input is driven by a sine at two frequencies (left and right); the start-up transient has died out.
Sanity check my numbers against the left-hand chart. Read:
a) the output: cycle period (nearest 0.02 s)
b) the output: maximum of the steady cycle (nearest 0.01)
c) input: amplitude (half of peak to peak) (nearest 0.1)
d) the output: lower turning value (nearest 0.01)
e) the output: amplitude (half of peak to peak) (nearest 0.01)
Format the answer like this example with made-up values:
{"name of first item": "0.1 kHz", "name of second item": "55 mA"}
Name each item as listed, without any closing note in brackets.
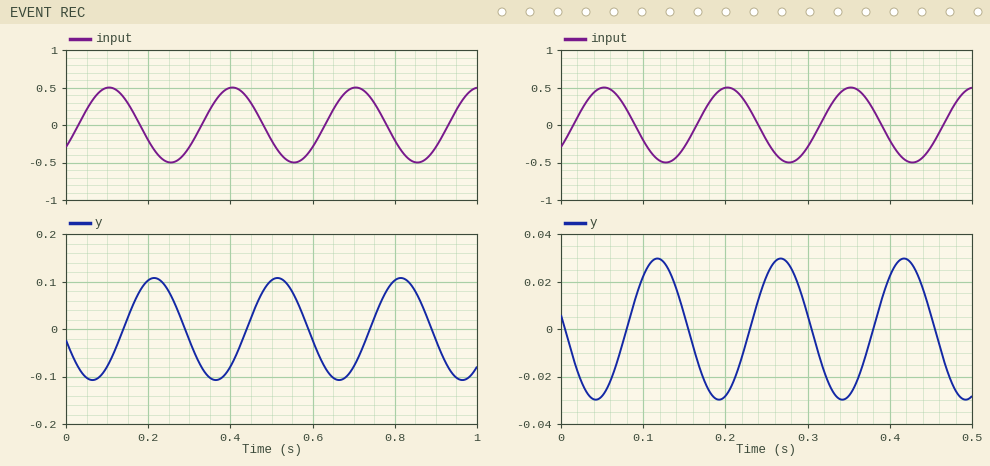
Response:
{"the output: cycle period": "0.30 s", "the output: maximum of the steady cycle": "0.11", "input: amplitude (half of peak to peak)": "0.5", "the output: lower turning value": "-0.11", "the output: amplitude (half of peak to peak)": "0.11"}
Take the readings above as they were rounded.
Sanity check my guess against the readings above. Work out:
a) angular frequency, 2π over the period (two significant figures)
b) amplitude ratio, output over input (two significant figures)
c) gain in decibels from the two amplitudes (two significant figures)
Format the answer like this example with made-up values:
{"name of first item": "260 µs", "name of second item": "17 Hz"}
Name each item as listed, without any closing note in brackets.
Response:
{"angular frequency, 2π over the period": "21 rad/s", "amplitude ratio, output over input": "0.22", "gain in decibels from the two amplitudes": "-13 dB"}
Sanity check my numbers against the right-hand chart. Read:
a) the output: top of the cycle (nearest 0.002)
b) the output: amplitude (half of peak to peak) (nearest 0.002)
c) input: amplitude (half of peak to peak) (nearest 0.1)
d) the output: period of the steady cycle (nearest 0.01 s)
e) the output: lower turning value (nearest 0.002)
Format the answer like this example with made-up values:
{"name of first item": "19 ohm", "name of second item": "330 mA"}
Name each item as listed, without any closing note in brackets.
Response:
{"the output: top of the cycle": "0.030", "the output: amplitude (half of peak to peak)": "0.030", "input: amplitude (half of peak to peak)": "0.5", "the output: period of the steady cycle": "0.15 s", "the output: lower turning value": "-0.030"}
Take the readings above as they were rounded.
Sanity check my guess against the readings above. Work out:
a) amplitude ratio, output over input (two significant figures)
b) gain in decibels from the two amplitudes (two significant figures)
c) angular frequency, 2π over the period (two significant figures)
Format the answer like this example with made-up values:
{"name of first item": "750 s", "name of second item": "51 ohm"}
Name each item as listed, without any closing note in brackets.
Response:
{"amplitude ratio, output over input": "0.060", "gain in decibels from the two amplitudes": "-24 dB", "angular frequency, 2π over the period": "42 rad/s"}
